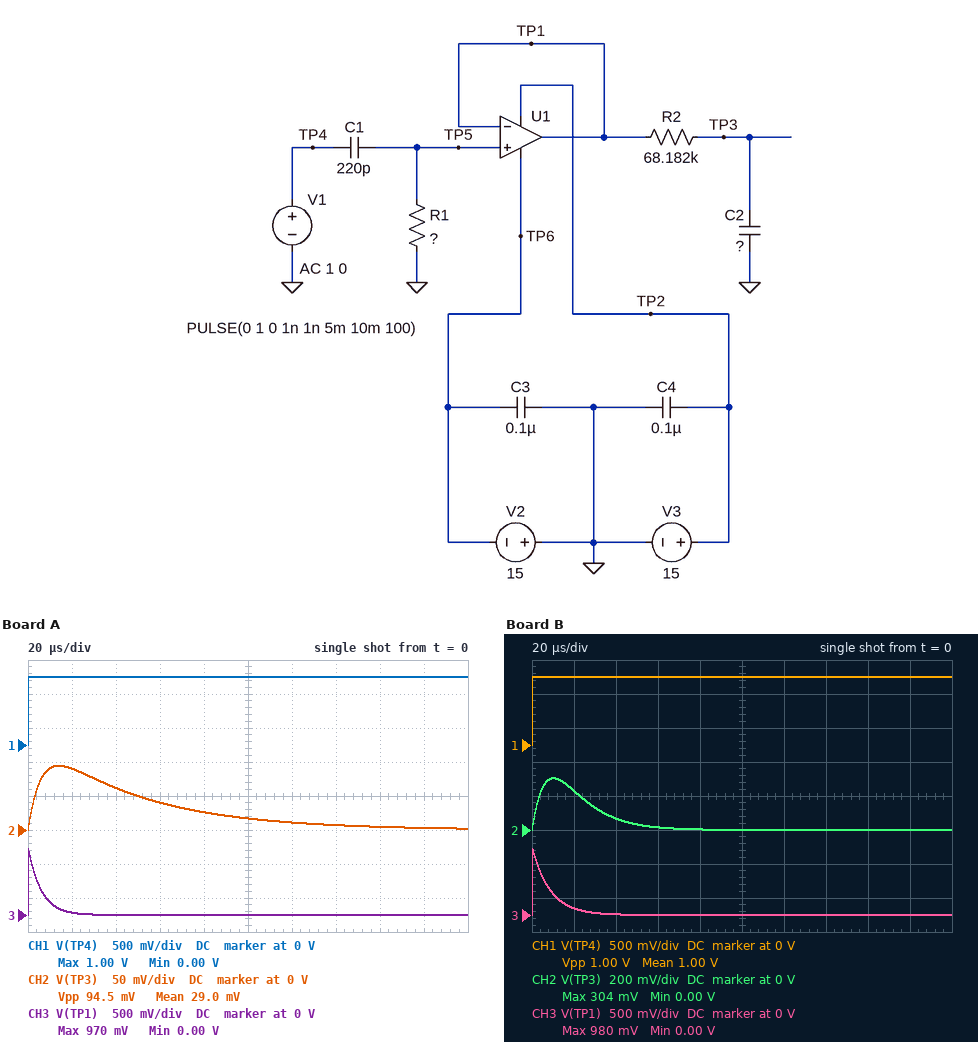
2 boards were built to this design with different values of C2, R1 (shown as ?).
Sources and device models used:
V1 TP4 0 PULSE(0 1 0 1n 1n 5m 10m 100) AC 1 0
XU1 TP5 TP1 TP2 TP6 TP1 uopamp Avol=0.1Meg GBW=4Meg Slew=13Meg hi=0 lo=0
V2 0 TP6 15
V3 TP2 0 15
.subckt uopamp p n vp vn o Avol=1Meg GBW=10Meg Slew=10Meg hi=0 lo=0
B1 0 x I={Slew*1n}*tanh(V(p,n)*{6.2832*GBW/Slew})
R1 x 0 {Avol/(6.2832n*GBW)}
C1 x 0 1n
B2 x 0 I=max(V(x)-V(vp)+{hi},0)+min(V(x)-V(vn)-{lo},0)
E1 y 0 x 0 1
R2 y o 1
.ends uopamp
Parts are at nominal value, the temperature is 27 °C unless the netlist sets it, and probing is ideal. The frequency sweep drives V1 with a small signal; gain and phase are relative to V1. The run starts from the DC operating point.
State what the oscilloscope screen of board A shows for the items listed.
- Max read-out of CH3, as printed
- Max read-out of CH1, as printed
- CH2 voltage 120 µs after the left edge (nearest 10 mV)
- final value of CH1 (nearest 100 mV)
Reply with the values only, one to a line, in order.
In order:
970 mV
1.00 V
10 mV
1.0 V
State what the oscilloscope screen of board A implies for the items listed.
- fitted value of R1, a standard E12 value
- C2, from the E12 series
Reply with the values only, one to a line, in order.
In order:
27 kΩ
680 pF
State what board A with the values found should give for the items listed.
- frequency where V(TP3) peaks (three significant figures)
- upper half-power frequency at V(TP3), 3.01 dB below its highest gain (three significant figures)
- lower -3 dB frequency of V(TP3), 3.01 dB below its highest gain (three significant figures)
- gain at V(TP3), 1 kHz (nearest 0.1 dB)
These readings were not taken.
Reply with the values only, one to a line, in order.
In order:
9.59 kHz
33.0 kHz
2.79 kHz
-28.9 dB
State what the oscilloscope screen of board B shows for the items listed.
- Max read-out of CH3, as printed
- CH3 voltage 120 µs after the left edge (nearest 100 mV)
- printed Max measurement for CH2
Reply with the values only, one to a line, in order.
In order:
980 mV
0 V
304 mV
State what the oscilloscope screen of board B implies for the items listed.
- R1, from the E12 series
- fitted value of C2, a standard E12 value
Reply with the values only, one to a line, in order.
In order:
39 kΩ
180 pF
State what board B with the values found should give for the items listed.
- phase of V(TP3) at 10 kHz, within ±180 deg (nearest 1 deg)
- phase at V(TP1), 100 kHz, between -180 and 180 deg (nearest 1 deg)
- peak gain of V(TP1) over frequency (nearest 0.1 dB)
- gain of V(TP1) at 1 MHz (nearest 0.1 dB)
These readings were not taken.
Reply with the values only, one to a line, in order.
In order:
24 deg
9 deg
0 dB
-0.3 dB
